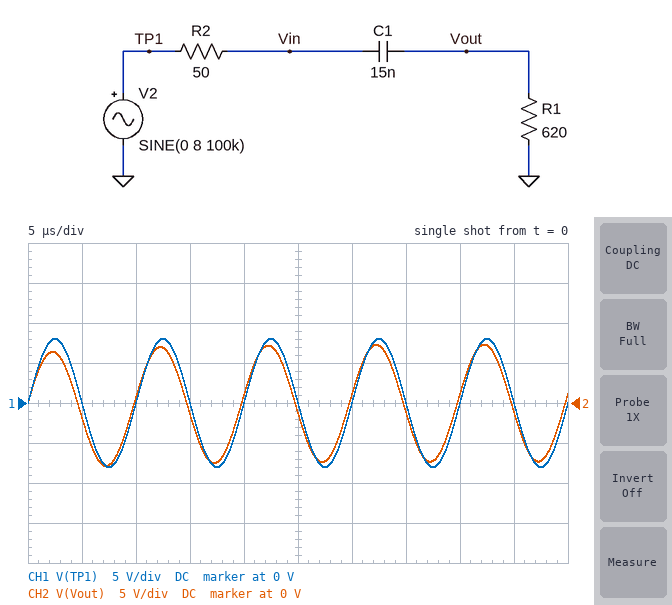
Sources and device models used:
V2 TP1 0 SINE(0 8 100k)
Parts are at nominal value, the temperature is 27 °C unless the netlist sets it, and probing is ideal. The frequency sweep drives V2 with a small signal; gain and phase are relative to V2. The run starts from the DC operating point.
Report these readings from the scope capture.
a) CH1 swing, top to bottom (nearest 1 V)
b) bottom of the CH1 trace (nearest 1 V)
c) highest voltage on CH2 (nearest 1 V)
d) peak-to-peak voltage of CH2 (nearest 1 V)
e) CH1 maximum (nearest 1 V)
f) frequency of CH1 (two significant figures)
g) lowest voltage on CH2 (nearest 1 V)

16 V
-8 V
7 V
15 V
8 V
100 kHz
-8 V
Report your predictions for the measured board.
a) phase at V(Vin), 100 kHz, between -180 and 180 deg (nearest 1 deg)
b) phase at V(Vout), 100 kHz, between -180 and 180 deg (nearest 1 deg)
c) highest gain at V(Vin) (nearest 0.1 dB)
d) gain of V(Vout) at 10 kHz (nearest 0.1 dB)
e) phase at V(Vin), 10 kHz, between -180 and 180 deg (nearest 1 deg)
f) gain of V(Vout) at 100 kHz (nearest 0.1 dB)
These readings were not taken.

-1 deg
9 deg
0 dB
-6.1 dB
-2 deg
-0.8 dB
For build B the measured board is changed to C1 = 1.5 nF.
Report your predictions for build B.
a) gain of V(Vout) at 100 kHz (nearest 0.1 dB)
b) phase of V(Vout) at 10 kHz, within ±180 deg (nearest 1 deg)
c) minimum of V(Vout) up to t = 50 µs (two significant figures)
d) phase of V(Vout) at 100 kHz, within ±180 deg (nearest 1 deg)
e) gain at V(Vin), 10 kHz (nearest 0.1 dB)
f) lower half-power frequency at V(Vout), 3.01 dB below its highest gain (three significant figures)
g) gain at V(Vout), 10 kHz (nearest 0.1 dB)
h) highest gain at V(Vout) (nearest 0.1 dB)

-6.1 dB
86 deg
-4.0 V
58 deg
0 dB
158 kHz
-24.7 dB
-0.7 dB
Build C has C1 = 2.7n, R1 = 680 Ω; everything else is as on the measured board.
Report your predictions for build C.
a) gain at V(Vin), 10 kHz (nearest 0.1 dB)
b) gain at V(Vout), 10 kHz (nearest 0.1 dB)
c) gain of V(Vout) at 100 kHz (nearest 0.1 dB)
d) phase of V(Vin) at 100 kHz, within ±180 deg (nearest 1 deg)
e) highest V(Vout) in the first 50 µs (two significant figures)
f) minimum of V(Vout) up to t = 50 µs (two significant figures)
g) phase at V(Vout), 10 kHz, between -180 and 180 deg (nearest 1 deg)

0 dB
-18.8 dB
-2.8 dB
-2 deg
5.8 V
-5.9 V
83 deg
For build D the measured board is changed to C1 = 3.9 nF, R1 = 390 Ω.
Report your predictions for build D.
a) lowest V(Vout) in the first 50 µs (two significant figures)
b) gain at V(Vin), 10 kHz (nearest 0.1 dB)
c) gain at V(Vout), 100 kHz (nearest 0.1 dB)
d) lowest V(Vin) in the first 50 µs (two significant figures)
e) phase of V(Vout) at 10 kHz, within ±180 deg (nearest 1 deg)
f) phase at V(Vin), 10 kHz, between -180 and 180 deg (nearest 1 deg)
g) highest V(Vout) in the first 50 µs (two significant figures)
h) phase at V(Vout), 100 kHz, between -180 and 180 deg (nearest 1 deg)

-5.3 V
0 dB
-3.7 dB
-7.5 V
84 deg
-1 deg
5.2 V
43 deg
